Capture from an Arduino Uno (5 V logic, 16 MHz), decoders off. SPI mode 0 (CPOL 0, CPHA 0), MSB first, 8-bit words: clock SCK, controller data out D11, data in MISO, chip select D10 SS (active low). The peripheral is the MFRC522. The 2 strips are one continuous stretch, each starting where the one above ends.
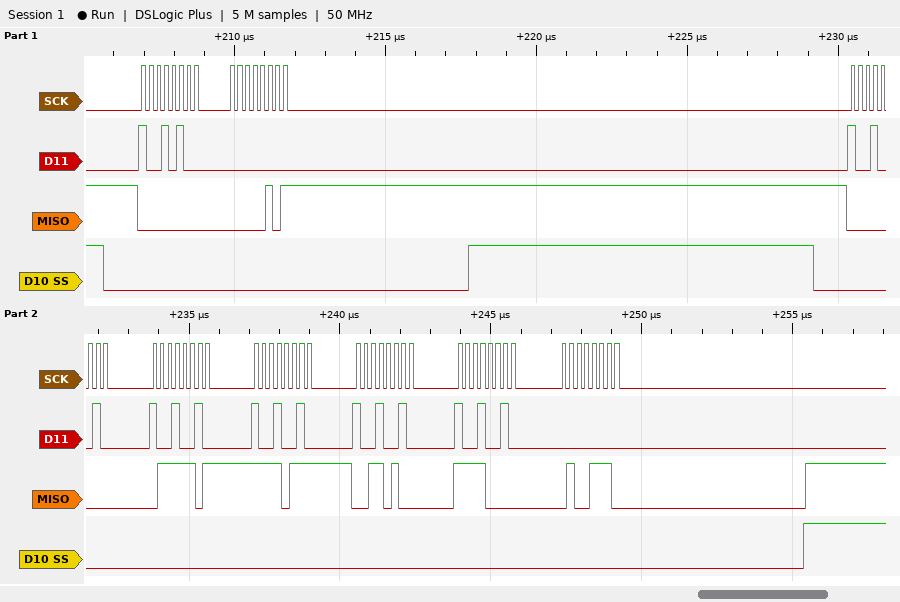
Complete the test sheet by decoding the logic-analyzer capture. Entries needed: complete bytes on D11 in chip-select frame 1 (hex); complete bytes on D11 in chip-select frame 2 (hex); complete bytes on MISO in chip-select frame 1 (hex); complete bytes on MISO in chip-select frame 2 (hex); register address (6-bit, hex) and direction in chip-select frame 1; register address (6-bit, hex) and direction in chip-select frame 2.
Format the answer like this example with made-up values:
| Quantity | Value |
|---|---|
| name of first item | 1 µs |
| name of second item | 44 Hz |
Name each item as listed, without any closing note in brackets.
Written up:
| Quantity | Value |
|---|---|
| complete bytes on D11 in chip-select frame 1 | 94 00 |
| complete bytes on D11 in chip-select frame 2 | 92 92 92 92 92 00 |
| complete bytes on MISO in chip-select frame 1 | 00 05 |
| complete bytes on MISO in chip-select frame 2 | 00 7D F7 34 F0 4E |
| register address (6-bit, hex) and direction in chip-select frame 1 | 0x0A read |
| register address (6-bit, hex) and direction in chip-select frame 2 | 0x09 read |
